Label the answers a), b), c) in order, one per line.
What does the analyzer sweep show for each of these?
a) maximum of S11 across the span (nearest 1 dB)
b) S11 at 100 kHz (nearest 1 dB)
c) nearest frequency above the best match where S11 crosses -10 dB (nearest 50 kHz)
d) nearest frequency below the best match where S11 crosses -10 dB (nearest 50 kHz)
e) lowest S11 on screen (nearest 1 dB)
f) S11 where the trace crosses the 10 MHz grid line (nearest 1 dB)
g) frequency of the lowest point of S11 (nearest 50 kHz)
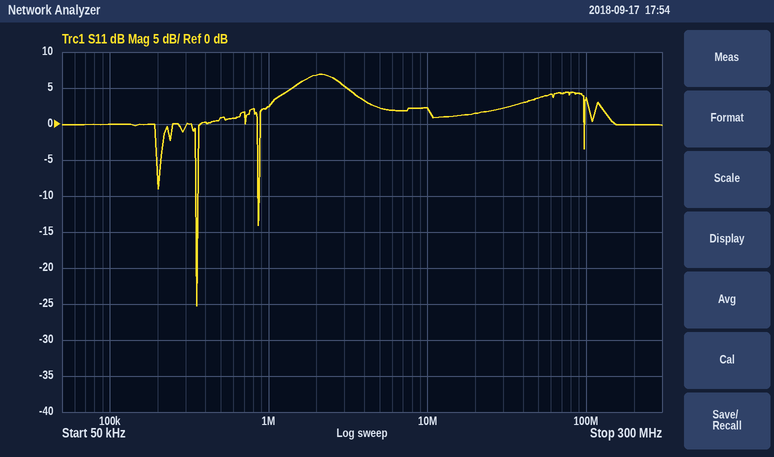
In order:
a) 7 dB
b) 0 dB
c) 350 kHz
d) 350 kHz
e) -25 dB
f) 2 dB
g) 350 kHz
